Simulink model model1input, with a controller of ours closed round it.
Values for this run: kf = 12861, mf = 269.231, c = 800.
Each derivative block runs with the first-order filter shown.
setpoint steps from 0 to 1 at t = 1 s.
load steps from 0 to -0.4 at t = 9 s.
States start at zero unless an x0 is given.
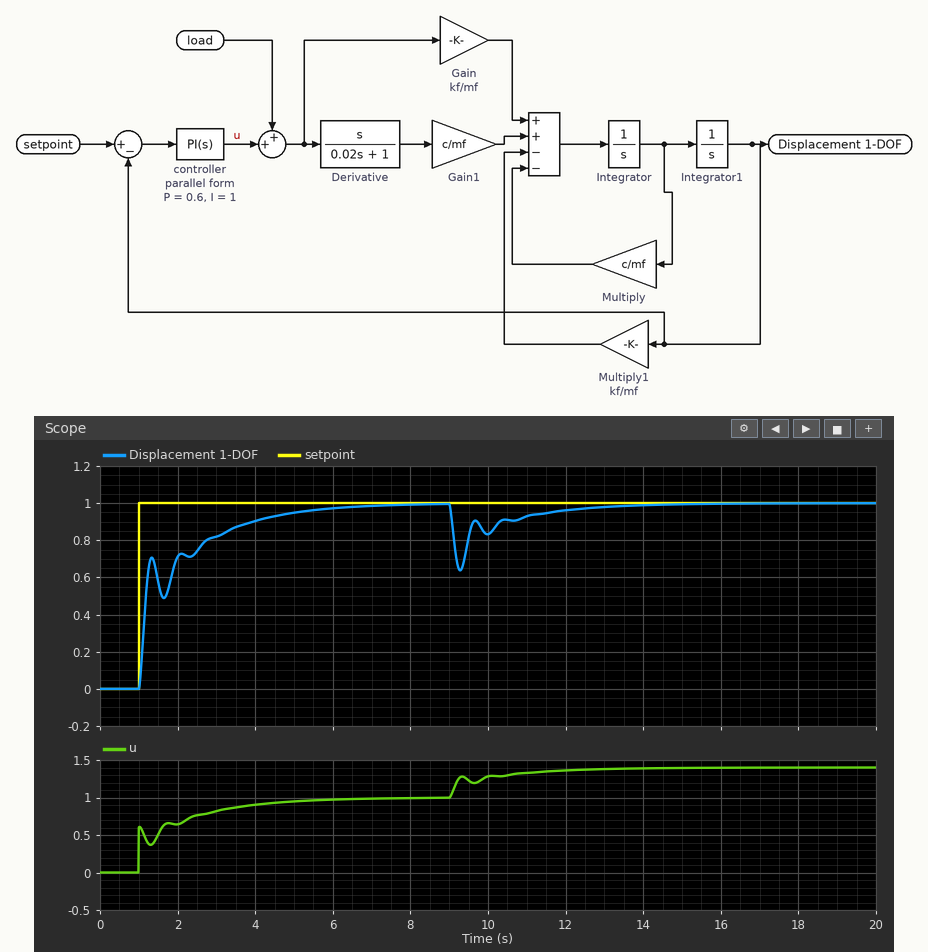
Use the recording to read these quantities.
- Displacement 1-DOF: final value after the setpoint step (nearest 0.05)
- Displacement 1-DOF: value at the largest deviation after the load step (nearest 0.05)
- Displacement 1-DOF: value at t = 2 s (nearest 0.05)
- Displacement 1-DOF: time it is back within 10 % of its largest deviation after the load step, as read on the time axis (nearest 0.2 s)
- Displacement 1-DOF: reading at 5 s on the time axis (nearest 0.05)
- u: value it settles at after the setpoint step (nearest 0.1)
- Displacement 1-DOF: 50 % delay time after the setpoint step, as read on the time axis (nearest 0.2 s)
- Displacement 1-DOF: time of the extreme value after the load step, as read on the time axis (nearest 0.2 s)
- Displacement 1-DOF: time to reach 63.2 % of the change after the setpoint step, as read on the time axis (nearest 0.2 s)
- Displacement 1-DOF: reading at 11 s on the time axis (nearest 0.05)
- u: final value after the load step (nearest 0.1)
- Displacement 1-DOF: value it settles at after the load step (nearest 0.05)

1.00
0.65
0.70
12.2 s
0.95
1.0
1.2 s
9.2 s
1.2 s
0.95
1.4
1.00
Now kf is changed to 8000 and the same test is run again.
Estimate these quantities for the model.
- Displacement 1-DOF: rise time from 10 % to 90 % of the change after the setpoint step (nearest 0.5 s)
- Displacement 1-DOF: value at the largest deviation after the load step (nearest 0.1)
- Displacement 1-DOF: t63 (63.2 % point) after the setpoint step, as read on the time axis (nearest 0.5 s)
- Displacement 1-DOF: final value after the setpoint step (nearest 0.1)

3.0 s
0.7
1.5 s
1.0
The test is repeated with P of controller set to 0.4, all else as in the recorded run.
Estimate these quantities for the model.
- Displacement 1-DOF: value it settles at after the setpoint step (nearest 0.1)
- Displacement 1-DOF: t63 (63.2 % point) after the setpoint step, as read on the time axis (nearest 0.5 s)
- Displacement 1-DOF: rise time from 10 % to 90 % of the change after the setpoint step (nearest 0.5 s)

1.0
2.0 s
2.5 s
